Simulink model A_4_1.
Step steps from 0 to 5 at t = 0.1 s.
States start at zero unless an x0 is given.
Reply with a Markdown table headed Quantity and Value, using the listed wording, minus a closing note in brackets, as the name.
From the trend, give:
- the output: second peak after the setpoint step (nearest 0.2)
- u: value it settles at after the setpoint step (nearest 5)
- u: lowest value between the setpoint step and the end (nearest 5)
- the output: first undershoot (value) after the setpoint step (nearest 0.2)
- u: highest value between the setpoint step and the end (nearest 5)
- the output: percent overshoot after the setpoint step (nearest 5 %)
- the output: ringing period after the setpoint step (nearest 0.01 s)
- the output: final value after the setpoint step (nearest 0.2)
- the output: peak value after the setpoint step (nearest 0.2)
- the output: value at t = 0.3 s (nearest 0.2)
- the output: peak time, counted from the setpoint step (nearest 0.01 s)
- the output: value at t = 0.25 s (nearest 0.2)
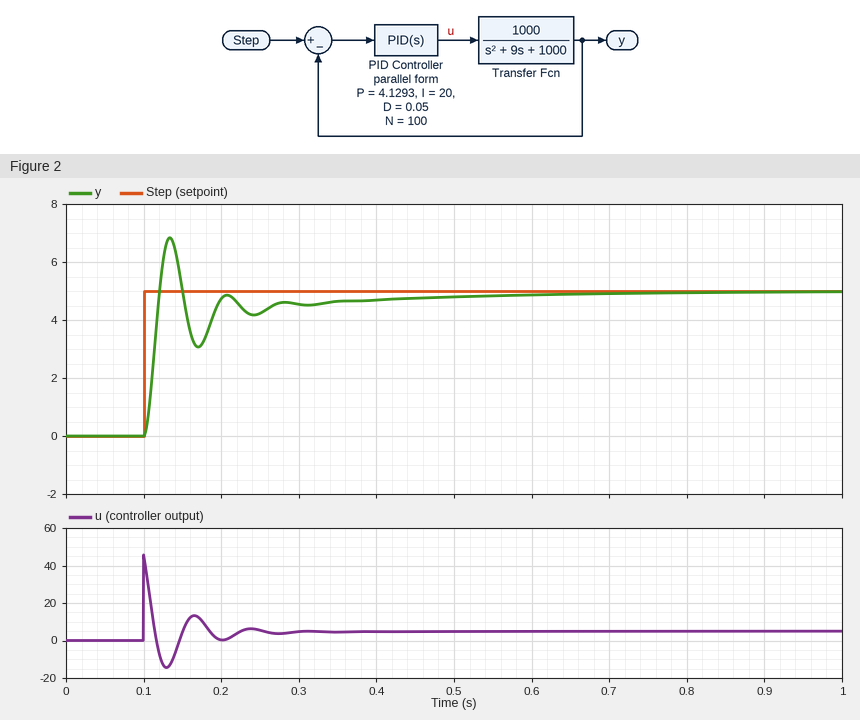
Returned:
| Quantity | Value |
|---|---|
| the output: second peak after the setpoint step | 4.8 |
| u: value it settles at after the setpoint step | 5 |
| u: lowest value between the setpoint step and the end | -15 |
| the output: first undershoot (value) after the setpoint step | 3.0 |
| u: highest value between the setpoint step and the end | 45 |
| the output: percent overshoot after the setpoint step | 35 % |
| the output: ringing period after the setpoint step | 0.07 s |
| the output: final value after the setpoint step | 5.0 |
| the output: peak value after the setpoint step | 6.8 |
| the output: value at t = 0.3 s | 4.6 |
| the output: peak time, counted from the setpoint step | 0.03 s |
| the output: value at t = 0.25 s | 4.2 |
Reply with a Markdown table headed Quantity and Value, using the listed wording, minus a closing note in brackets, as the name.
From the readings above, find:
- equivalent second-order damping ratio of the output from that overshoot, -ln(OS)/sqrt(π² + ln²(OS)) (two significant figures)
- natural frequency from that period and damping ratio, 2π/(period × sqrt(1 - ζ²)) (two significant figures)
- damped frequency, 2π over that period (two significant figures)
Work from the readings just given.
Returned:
| Quantity | Value |
|---|---|
| equivalent second-order damping ratio of the output from that overshoot, -ln(OS)/sqrt(π² + ln²(OS)) | 0.32 |
| natural frequency from that period and damping ratio, 2π/(period × sqrt(1 - ζ²)) | 95 rad/s |
| damped frequency, 2π over that period | 90 rad/s |
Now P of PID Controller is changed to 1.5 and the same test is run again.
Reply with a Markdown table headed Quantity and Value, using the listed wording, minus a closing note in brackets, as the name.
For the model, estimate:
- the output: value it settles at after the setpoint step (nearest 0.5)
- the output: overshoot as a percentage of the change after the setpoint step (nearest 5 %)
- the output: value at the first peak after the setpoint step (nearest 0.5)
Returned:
| Quantity | Value |
|---|---|
| the output: value it settles at after the setpoint step | 5.0 |
| the output: overshoot as a percentage of the change after the setpoint step | 10 % |
| the output: value at the first peak after the setpoint step | 5.5 |
